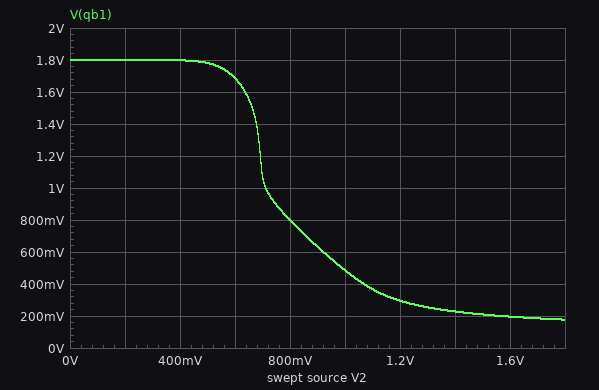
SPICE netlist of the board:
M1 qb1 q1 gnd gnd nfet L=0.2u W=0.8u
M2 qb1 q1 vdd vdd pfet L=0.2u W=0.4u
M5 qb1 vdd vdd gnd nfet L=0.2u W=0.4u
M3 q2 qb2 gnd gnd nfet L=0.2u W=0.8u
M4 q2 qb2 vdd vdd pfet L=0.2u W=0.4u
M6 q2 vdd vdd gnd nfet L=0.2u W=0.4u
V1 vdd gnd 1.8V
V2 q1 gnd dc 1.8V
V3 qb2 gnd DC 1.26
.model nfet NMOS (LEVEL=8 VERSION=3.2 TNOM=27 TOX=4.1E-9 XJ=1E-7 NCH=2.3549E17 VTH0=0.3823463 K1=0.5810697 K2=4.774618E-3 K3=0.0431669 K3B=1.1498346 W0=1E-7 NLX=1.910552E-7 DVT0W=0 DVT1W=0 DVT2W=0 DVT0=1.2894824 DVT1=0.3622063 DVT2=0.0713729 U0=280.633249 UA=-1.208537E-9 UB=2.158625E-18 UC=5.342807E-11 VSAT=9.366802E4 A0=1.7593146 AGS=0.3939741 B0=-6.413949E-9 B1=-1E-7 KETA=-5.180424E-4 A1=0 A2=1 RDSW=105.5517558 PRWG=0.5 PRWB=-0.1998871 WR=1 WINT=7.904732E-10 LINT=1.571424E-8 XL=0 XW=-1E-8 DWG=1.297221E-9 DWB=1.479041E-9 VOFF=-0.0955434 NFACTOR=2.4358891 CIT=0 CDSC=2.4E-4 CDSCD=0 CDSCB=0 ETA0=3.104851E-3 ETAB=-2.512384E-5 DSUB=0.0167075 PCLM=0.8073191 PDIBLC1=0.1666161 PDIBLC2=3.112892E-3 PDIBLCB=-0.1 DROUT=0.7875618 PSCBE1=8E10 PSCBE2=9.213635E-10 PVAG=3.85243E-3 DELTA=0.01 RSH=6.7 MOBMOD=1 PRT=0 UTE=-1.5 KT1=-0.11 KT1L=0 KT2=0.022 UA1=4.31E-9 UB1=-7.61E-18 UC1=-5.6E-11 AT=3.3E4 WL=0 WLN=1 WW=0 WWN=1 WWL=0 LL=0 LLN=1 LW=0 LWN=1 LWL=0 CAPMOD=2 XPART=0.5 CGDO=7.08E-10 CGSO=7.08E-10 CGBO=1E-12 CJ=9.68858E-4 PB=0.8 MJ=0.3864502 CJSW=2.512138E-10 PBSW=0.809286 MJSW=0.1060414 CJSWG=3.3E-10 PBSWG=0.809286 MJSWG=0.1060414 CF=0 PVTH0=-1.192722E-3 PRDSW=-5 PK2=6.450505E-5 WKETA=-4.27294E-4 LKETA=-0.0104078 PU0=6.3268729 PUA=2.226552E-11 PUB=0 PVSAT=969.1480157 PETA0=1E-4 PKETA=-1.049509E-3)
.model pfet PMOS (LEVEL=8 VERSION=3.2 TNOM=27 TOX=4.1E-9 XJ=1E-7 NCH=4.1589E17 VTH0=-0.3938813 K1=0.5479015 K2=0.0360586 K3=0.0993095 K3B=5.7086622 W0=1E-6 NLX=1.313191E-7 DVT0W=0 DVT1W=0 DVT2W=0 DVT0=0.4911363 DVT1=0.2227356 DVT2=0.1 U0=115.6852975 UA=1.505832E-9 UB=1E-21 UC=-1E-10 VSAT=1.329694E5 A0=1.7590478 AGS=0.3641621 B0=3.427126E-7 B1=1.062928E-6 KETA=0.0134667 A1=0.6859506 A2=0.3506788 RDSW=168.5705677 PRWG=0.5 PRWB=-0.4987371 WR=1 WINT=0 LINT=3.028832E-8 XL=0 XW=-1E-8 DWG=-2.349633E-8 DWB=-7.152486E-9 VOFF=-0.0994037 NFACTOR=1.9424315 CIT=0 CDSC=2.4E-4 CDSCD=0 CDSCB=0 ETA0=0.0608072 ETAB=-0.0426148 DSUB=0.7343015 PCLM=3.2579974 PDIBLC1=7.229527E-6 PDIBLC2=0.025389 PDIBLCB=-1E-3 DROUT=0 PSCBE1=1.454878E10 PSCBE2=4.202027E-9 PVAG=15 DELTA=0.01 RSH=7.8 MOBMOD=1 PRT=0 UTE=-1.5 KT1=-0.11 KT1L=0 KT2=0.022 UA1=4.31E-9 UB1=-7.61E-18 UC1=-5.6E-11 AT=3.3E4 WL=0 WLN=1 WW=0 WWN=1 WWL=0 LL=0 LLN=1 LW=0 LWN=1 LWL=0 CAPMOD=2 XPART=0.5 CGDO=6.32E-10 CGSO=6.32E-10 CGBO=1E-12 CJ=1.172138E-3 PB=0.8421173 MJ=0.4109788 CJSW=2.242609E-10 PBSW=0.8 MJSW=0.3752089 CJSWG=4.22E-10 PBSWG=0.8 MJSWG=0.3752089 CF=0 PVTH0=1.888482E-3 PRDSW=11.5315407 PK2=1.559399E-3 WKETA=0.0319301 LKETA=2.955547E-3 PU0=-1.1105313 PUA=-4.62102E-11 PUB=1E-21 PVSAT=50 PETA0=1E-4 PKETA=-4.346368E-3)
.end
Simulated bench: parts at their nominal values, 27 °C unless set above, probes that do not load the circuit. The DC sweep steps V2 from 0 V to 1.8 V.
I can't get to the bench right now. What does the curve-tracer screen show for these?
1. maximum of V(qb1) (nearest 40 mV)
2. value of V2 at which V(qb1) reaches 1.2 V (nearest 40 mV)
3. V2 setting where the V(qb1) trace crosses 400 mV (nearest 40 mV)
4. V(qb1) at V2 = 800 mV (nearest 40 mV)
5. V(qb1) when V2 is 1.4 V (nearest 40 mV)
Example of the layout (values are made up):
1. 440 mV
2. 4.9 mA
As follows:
1. 1.80 V
2. 680 mV
3. 1.08 V
4. 800 mV
5. 240 mV
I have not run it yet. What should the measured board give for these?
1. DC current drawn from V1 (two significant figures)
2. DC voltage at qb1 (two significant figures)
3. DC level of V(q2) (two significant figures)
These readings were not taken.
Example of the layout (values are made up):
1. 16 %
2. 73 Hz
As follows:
1. 340 µA
2. 180 mV
3. 290 mV
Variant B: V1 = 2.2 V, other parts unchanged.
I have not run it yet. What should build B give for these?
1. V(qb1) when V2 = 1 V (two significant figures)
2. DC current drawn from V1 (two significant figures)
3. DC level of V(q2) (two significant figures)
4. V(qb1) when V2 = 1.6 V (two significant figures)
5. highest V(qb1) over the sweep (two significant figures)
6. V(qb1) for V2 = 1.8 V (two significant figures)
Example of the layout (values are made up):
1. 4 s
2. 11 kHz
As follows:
1. 910 mV
2. 440 µA
3. 560 mV
4. 300 mV
5. 2.2 V
6. 260 mV
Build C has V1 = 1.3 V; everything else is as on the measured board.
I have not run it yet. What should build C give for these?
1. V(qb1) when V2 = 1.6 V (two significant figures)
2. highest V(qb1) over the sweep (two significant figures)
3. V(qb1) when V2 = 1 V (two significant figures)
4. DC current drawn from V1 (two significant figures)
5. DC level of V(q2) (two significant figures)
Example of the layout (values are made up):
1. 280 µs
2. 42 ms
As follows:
1. 94 mV
2. 1.3 V
3. 170 mV
4. 190 µA
5. 130 mV
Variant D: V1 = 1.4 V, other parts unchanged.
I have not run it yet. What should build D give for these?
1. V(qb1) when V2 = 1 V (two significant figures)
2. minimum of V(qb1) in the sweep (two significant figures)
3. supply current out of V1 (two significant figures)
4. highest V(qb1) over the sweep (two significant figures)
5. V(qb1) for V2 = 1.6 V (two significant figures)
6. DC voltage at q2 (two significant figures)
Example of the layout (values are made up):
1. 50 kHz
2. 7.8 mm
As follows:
1. 210 mV
2. 100 mV
3. 220 µA
4. 1.4 V
5. 110 mV
6. 160 mV
